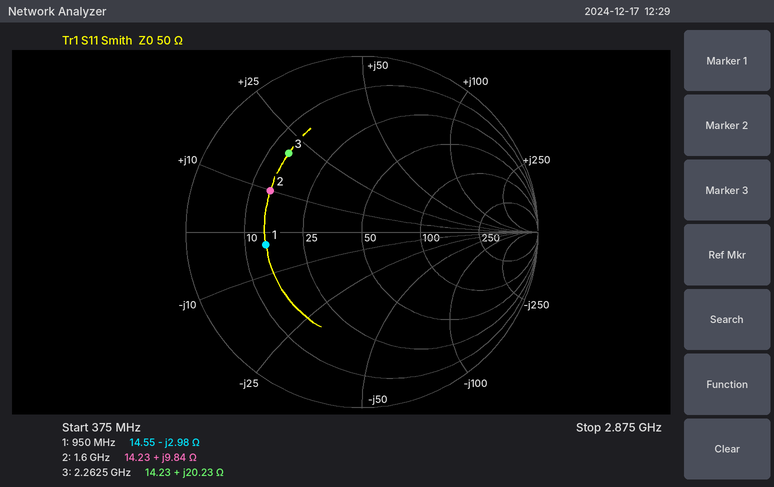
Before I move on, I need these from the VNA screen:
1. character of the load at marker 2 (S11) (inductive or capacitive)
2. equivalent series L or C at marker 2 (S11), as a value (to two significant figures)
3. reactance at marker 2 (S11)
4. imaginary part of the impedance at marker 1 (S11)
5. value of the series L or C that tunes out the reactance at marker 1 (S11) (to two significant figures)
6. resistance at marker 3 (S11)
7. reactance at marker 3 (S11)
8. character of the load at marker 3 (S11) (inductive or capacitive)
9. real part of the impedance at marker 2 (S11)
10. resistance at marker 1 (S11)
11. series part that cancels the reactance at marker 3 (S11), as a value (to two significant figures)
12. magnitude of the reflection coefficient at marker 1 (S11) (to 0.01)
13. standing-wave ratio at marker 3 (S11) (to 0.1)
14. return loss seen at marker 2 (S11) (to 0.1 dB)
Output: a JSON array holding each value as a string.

["inductive", "980 pH", "+9.84 Ω", "-2.98 Ω", "500 pH", "14.23 Ω", "+20.23 Ω", "inductive", "14.23 Ω", "14.55 Ω", "3.5 pF", "0.55", "4.1", "4.9 dB"]
